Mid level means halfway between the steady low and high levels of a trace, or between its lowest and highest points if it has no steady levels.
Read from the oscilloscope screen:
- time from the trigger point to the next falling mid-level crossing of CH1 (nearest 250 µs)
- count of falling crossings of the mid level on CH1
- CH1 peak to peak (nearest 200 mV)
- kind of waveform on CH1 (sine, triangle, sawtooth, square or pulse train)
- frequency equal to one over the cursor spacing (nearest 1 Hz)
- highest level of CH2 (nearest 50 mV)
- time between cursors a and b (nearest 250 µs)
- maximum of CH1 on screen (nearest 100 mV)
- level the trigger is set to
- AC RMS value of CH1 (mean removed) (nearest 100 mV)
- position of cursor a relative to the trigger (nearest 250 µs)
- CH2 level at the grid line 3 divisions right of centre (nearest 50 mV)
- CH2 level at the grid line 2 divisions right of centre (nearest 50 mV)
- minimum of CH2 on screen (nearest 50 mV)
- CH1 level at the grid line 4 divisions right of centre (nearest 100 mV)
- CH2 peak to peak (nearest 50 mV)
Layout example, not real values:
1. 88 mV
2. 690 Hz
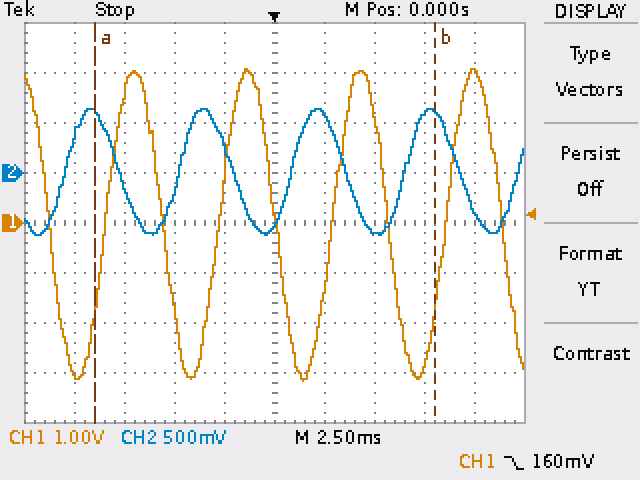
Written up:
1. 5.75 ms
2. 5
3. 6.2 V
4. sine
5. 59 Hz
6. 650 mV
7. 17.00 ms
8. 3.1 V
9. 160 mV
10. 2.2 V
11. -9.00 ms
12. 600 mV
13. -600 mV
14. -600 mV
15. 3.0 V
16. 1.25 V
